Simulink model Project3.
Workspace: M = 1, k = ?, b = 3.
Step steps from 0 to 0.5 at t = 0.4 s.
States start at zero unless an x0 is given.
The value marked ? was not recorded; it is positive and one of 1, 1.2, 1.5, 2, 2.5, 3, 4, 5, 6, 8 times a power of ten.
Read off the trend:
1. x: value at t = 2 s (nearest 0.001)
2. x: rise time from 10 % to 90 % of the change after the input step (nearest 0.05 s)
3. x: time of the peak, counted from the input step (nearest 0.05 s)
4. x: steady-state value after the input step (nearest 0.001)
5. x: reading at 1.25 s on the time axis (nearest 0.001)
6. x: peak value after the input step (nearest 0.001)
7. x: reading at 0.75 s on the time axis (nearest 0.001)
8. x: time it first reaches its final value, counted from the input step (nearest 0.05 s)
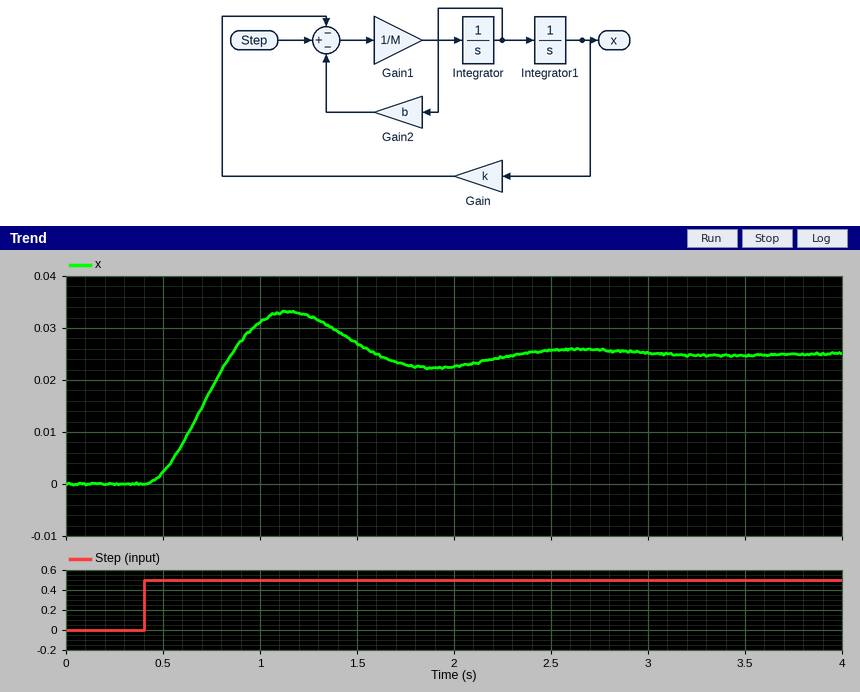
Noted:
0.023
0.30 s
0.75 s
0.025
0.032
0.033
0.018
0.45 s
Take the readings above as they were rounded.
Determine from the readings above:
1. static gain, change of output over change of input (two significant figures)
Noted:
0.050
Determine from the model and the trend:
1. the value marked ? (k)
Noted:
20
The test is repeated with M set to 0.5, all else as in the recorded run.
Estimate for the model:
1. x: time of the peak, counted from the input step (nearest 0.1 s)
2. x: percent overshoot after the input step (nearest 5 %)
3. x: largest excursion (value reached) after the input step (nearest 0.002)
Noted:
0.6 s
20 %
0.030
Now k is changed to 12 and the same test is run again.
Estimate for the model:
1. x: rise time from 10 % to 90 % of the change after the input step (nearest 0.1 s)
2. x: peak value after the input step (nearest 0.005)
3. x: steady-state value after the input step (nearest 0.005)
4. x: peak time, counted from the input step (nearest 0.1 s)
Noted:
0.4 s
0.050
0.040
1.0 s
